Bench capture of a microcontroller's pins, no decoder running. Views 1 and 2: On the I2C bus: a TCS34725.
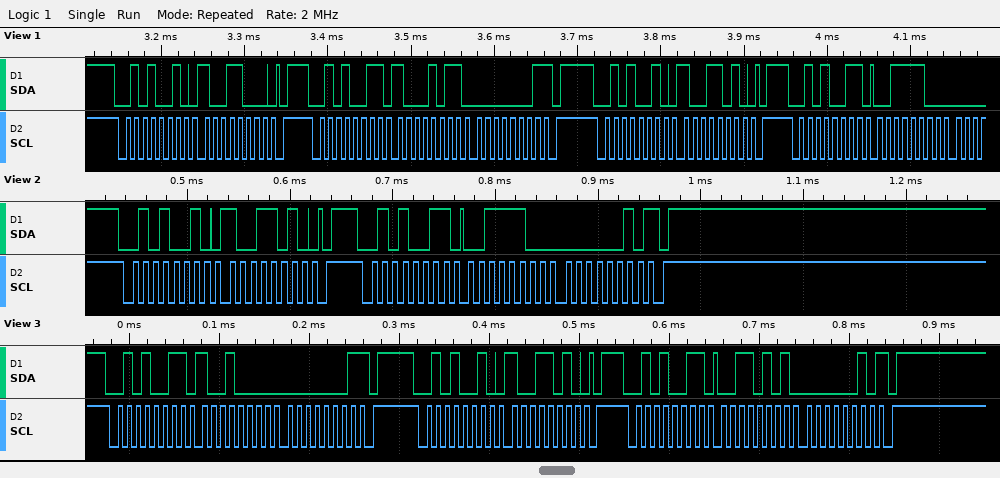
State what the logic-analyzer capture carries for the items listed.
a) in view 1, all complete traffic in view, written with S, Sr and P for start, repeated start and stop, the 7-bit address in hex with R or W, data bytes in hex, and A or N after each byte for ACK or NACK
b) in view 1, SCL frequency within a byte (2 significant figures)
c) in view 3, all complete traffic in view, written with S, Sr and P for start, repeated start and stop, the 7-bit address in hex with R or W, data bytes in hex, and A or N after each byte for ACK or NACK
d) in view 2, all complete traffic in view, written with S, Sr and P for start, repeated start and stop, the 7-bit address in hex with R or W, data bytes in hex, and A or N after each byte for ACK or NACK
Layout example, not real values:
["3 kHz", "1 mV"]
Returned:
["S 29W A 98 A P S 29R A 8B A 01 N P S 29W A 9A A P S 29R A 3C A", "100 kHz", "S 29R A 90 A 01 N P S 29W A 9A A P S 29R A 35 A 02 N P", "S 29W A 9A A P S 29R A 3C A 02 N P"]
